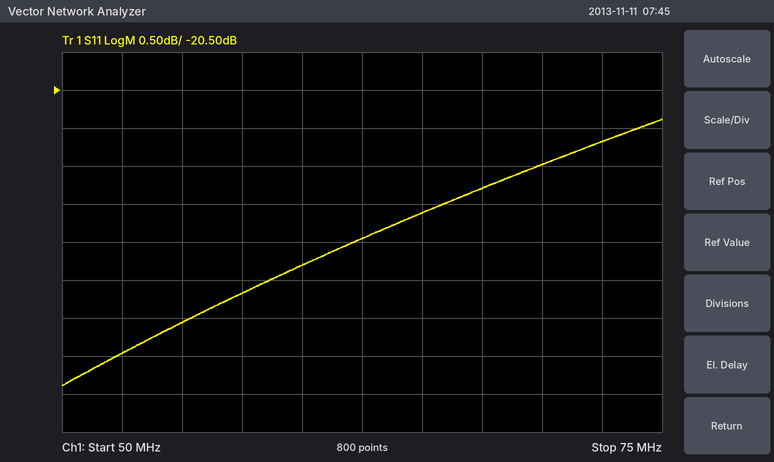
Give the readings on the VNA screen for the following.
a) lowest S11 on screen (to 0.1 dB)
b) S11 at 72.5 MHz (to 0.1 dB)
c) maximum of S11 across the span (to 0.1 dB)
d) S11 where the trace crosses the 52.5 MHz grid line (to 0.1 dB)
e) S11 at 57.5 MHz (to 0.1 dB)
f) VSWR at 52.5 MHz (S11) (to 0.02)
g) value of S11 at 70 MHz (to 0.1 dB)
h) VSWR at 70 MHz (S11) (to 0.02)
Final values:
-24.4 dB
-21.2 dB
-20.9 dB
-24.0 dB
-23.2 dB
1.14
-21.5 dB
1.18
